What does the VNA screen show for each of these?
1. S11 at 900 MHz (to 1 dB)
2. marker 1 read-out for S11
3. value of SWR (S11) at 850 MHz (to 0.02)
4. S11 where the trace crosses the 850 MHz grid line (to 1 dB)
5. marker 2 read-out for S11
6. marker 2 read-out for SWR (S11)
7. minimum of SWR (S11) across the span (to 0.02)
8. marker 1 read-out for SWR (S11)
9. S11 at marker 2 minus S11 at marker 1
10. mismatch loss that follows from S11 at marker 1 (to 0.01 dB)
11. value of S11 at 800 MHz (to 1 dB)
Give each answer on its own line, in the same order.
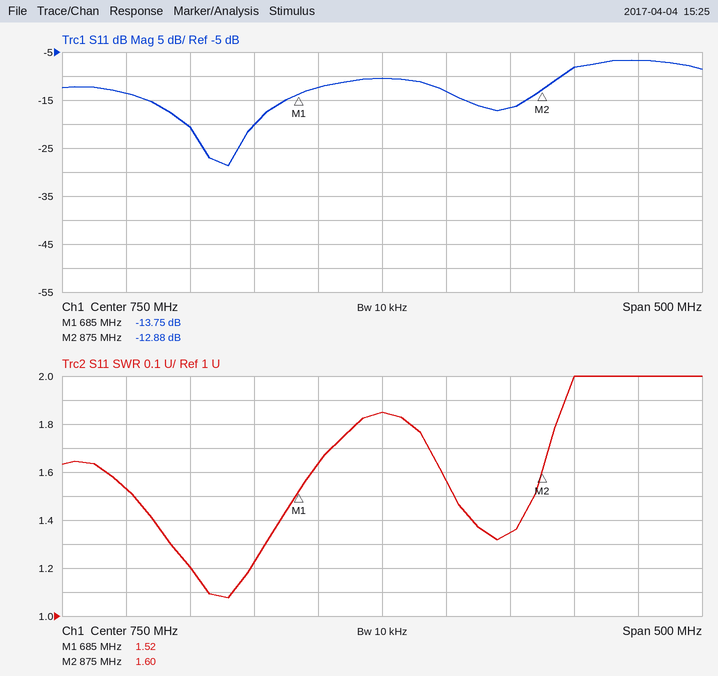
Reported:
-8 dB
-13.75 dB
1.34
-17 dB
-12.88 dB
1.60
1.08
1.52
0.87 dB
0.19 dB
-13 dB
